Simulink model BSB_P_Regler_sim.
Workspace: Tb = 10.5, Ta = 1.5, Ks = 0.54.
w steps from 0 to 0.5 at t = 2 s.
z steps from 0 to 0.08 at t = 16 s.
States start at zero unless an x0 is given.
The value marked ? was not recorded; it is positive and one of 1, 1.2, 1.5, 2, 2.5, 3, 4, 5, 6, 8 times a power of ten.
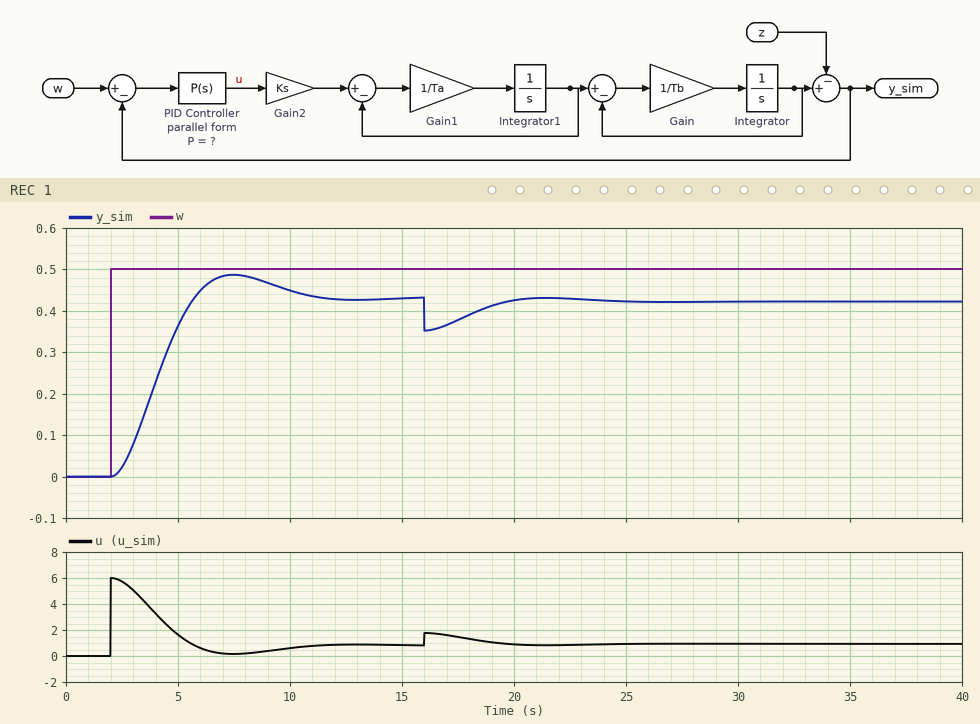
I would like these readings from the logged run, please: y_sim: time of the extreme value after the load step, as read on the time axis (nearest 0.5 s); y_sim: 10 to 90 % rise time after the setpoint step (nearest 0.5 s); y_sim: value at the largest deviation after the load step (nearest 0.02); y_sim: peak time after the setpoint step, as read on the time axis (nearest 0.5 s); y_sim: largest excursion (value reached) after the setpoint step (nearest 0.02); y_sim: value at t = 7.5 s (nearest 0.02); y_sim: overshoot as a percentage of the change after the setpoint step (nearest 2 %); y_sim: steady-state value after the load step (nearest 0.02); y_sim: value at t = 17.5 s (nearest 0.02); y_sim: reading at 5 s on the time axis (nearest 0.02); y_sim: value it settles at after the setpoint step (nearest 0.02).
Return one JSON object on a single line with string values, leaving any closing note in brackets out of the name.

{"y_sim: time of the extreme value after the load step, as read on the time axis": "16.0 s", "y_sim: 10 to 90 % rise time after the setpoint step": "2.5 s", "y_sim: value at the largest deviation after the load step": "0.36", "y_sim: peak time after the setpoint step, as read on the time axis": "7.5 s", "y_sim: largest excursion (value reached) after the setpoint step": "0.48", "y_sim: value at t = 7.5 s": "0.48", "y_sim: overshoot as a percentage of the change after the setpoint step": "12 %", "y_sim: steady-state value after the load step": "0.42", "y_sim: value at t = 17.5 s": "0.38", "y_sim: reading at 5 s on the time axis": "0.36", "y_sim: value it settles at after the setpoint step": "0.44"}
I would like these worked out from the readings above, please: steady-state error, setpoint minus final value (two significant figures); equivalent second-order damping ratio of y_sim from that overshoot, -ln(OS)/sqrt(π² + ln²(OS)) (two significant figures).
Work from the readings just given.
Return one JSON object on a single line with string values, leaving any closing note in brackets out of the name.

{"steady-state error, setpoint minus final value": "0.060", "equivalent second-order damping ratio of y_sim from that overshoot, -ln(OS)/sqrt(π² + ln²(OS))": "0.56"}
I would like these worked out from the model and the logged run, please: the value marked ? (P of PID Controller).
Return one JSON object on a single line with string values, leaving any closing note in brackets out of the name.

{"the value marked ?": "12"}
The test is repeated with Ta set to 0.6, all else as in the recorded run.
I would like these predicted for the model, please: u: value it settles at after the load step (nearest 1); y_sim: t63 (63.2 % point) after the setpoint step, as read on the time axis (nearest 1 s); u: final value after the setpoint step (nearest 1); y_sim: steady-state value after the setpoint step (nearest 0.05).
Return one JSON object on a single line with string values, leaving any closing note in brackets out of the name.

{"u: value it settles at after the load step": "1", "y_sim: t63 (63.2 % point) after the setpoint step, as read on the time axis": "4 s", "u: final value after the setpoint step": "1", "y_sim: steady-state value after the setpoint step": "0.45"}
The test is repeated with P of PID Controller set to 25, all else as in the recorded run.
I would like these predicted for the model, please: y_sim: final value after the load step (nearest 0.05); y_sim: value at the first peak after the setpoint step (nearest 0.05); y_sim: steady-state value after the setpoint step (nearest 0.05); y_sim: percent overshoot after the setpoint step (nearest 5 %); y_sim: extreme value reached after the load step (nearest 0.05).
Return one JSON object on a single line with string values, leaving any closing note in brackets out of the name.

{"y_sim: final value after the load step": "0.45", "y_sim: value at the first peak after the setpoint step": "0.60", "y_sim: steady-state value after the setpoint step": "0.45", "y_sim: percent overshoot after the setpoint step": "25 %", "y_sim: extreme value reached after the load step": "0.40"}
